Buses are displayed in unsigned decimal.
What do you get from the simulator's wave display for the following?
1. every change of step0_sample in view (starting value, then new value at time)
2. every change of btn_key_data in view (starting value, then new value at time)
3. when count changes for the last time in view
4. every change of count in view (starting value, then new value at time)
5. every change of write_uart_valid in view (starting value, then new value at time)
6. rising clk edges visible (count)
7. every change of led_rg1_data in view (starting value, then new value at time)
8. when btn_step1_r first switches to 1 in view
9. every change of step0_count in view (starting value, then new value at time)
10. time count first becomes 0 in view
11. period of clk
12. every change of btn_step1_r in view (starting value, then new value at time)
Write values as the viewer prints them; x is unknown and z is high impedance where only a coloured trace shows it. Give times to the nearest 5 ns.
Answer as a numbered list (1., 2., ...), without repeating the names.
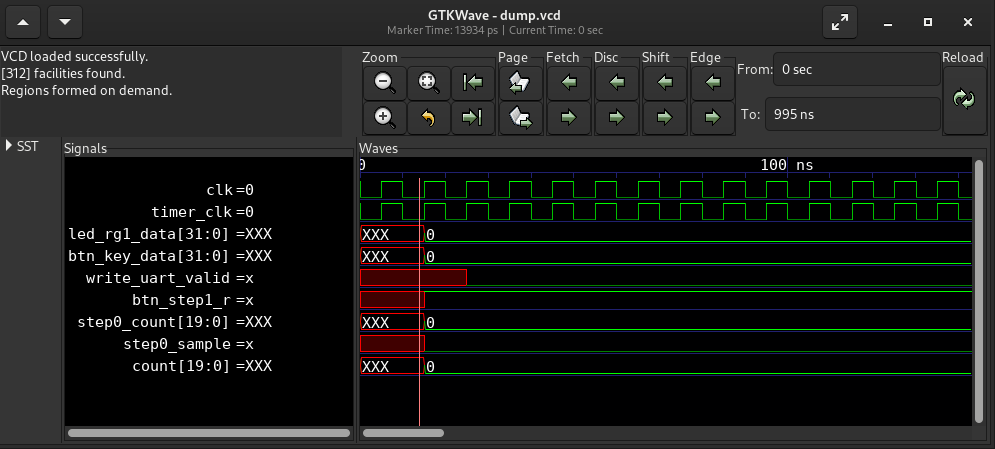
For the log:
1. x, 0 at 15 ns
2. XXX, 0 at 15 ns
3. 15 ns
4. XXX, 0 at 15 ns
5. x, 0 at 25 ns
6. 14
7. XXX, 0 at 15 ns
8. 15 ns
9. XXX, 0 at 15 ns
10. 15 ns
11. 10 ns
12. x, 1 at 15 ns
